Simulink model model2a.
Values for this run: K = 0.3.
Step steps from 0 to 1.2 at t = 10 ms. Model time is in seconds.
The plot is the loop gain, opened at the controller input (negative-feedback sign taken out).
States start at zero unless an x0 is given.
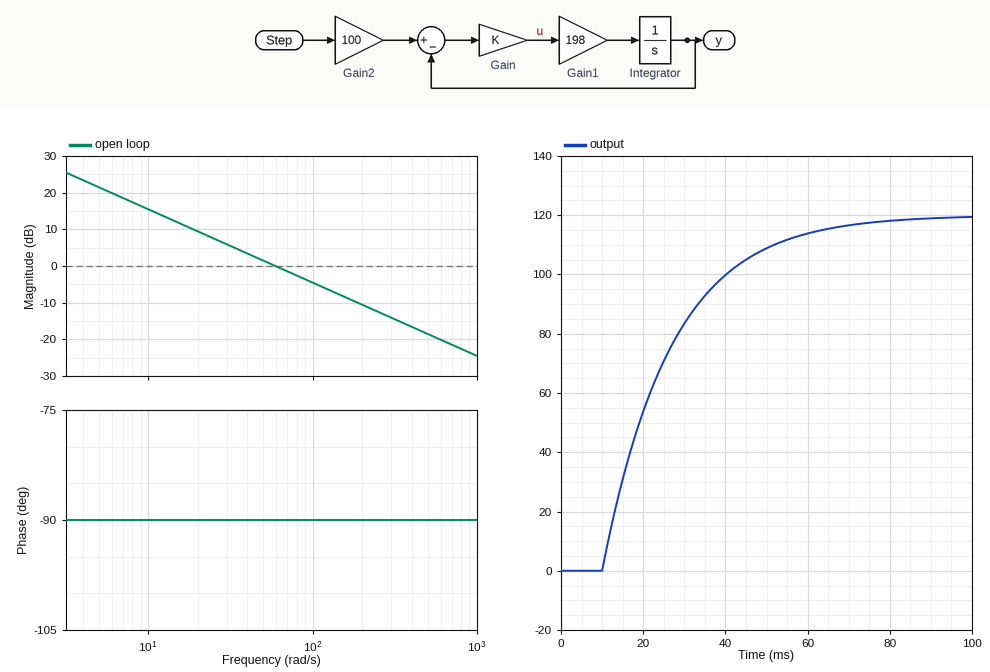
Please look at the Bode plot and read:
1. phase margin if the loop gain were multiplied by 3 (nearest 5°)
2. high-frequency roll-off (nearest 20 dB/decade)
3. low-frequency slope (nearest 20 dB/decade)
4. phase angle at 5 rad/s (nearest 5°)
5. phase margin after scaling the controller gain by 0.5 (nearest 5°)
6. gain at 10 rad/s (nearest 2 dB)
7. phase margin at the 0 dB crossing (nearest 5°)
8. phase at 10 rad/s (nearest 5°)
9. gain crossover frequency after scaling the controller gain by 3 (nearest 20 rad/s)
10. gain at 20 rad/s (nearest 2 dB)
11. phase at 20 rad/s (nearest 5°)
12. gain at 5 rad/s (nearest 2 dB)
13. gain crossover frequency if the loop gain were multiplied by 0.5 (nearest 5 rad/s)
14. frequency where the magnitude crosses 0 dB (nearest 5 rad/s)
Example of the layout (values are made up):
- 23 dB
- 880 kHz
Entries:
- 90°
- -20 dB/decade
- -20 dB/decade
- -90°
- 90°
- 16 dB
- 90°
- -90°
- 180 rad/s
- 10 dB
- -90°
- 22 dB
- 30 rad/s
- 60 rad/s
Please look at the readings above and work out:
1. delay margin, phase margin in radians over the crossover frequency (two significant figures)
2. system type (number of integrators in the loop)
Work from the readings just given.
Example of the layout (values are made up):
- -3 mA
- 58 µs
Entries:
- 0.026 s
- 1
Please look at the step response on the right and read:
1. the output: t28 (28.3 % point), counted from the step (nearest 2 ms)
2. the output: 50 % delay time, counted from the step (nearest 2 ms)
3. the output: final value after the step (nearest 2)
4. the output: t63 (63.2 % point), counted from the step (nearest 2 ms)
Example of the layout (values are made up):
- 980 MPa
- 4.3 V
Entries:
- 6 ms
- 12 ms
- 120
- 16 ms
